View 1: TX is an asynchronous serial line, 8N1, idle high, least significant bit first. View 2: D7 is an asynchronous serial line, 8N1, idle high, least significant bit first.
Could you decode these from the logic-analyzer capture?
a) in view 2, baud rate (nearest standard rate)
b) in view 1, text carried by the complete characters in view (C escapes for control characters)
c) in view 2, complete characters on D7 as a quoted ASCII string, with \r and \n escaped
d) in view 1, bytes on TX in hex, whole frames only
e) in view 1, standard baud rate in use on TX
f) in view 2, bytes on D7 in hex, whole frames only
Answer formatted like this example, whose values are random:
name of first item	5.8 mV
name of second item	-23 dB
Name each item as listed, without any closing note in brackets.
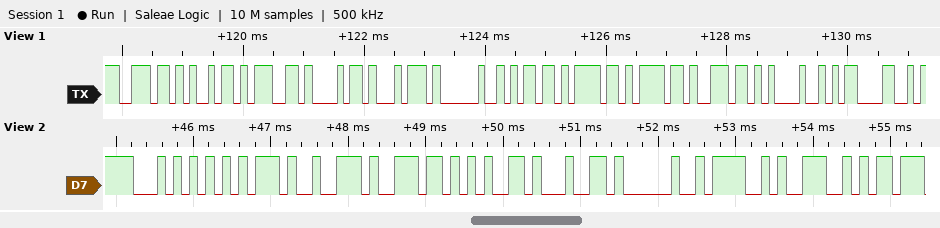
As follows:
in view 2, baud rate	9600 baud
in view 1, text carried by the complete characters in view	"night moon!\r"
in view 2, complete characters on D7 as a quoted ASCII string, with \r and \n escaped	"Turned ON"
in view 1, bytes on TX in hex, whole frames only	6E 69 67 68 74 20 6D 6F 6F 6E 21 0D
in view 1, standard baud rate in use on TX	9600 baud
in view 2, bytes on D7 in hex, whole frames only	54 75 72 6E 65 64 20 4F 4E
